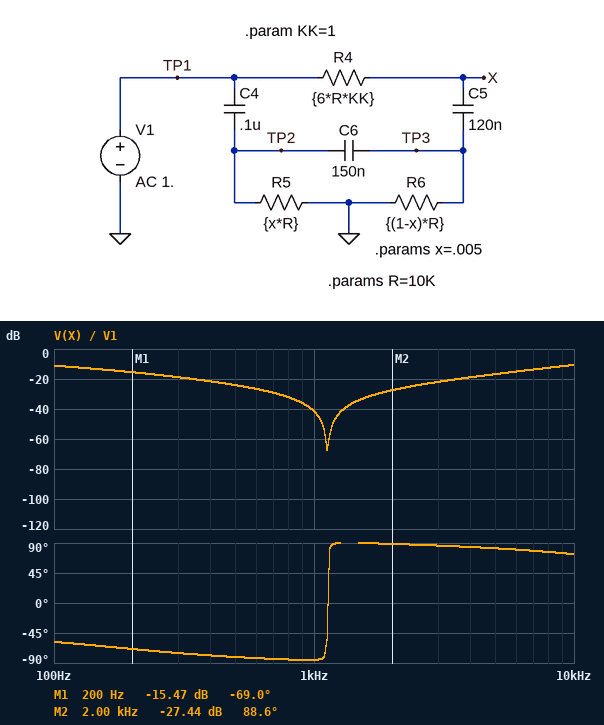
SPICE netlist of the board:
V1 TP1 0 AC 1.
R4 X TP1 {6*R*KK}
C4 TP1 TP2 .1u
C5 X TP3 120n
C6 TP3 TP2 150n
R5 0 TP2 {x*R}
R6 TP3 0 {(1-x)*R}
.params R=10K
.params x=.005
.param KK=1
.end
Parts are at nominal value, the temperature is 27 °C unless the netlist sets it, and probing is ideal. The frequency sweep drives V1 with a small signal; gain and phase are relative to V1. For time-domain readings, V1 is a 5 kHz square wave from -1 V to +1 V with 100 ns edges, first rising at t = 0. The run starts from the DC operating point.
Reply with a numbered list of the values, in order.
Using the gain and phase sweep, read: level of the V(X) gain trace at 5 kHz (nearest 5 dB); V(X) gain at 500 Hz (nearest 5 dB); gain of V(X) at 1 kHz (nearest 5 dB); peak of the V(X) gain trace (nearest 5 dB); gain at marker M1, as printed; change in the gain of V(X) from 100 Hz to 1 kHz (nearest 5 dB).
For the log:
1. -15 dB
2. -25 dB
3. -40 dB
4. -10 dB
5. -15.47 dB
6. -30 dB
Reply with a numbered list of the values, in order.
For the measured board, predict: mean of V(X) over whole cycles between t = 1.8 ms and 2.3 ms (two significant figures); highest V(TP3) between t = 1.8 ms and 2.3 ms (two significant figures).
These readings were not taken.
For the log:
1. -650 mV
2. 2.1 V
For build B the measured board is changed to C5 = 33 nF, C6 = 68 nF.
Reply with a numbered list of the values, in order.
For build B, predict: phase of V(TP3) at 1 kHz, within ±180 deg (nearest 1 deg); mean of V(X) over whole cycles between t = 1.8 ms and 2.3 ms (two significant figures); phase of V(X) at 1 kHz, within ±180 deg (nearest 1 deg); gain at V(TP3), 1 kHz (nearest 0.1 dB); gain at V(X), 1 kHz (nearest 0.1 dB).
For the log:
1. -41 deg
2. -310 mV
3. -81 deg
4. -41.5 dB
5. -21.3 dB
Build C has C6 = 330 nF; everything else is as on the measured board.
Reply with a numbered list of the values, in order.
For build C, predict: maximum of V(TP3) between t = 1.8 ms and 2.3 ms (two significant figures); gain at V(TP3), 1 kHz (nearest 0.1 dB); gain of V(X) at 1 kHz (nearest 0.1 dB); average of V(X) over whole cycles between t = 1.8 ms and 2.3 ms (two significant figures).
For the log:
1. 2.0 V
2. -32.7 dB
3. -57.6 dB
4. -700 mV
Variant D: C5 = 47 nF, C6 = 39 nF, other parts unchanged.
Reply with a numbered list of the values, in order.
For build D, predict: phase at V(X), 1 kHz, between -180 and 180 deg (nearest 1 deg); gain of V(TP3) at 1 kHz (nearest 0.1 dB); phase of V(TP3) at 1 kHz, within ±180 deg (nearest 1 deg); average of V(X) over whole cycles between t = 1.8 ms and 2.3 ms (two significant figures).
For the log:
1. -74 deg
2. -29.6 dB
3. -56 deg
4. -450 mV
